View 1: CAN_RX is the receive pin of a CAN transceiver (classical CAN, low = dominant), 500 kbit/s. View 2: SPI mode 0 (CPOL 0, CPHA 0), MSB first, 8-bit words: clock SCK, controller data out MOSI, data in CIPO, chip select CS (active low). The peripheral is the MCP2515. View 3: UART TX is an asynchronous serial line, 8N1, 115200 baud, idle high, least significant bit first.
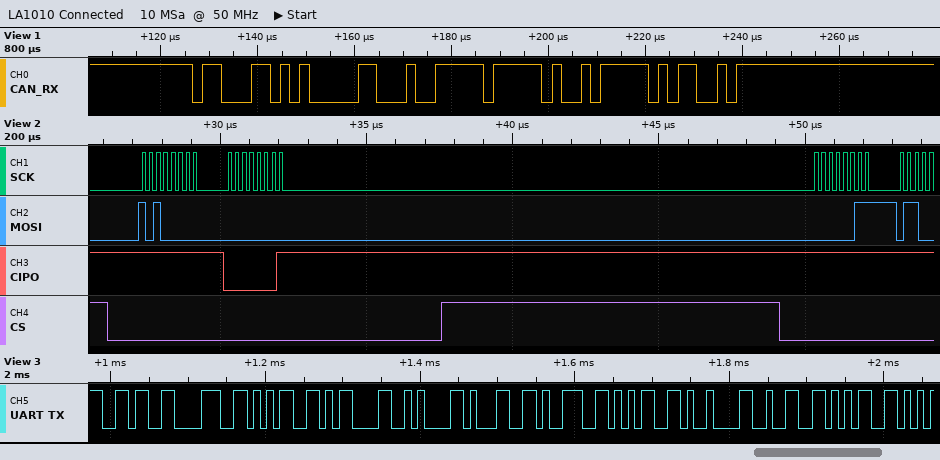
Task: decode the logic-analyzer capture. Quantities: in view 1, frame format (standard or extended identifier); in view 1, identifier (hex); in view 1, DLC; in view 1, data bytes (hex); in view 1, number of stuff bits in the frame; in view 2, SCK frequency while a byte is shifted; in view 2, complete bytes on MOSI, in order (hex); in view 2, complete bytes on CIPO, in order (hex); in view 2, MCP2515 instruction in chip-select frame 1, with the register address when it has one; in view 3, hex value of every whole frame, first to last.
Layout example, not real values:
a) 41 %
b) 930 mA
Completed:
a) standard
b) 0x635
c) 2
d) 27 FF
e) 4
f) 4 MHz
g) A0 00 03
h) FF 01 FF
i) READ STATUS
j) 0x36 0x38 0x35 0x0D 0x0A 0x31 0x39 0x35 0x09 0x32 0x35
